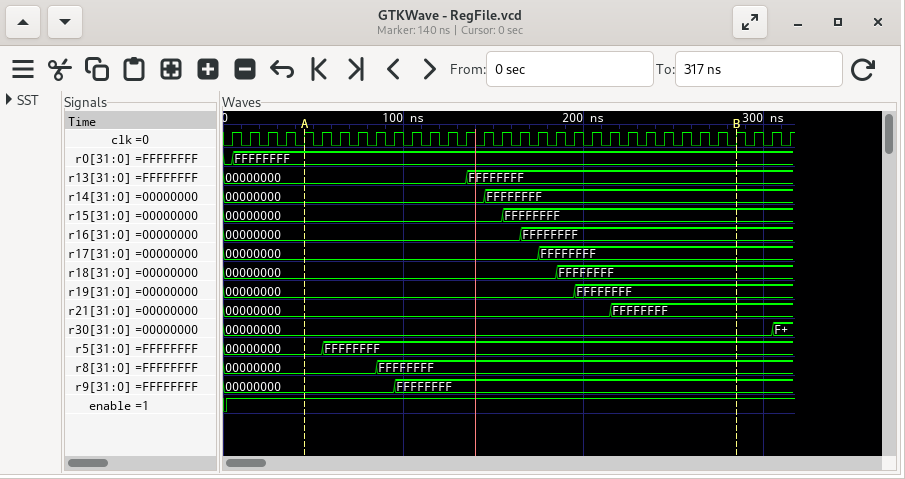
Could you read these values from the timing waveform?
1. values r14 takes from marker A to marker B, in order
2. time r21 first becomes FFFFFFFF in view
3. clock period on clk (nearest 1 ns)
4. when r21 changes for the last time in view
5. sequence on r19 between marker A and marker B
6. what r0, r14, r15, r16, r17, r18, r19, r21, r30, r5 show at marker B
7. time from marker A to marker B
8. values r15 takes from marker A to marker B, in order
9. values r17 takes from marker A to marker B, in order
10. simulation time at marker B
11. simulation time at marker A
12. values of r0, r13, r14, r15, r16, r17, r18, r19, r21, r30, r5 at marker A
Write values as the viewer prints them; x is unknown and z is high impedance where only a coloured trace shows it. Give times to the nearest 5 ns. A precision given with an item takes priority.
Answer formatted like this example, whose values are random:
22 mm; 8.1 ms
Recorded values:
00000000, FFFFFFFF; 215 ns; 10 ns; 215 ns; 00000000, FFFFFFFF; r0=FFFFFFFF, r14=FFFFFFFF, r15=FFFFFFFF, r16=FFFFFFFF, r17=FFFFFFFF, r18=FFFFFFFF, r19=FFFFFFFF, r21=FFFFFFFF, r30=00000000, r5=FFFFFFFF; 240 ns; 00000000, FFFFFFFF; 00000000, FFFFFFFF; 285 ns; 45 ns; r0=FFFFFFFF, r13=00000000, r14=00000000, r15=00000000, r16=00000000, r17=00000000, r18=00000000, r19=00000000, r21=00000000, r30=00000000, r5=00000000
